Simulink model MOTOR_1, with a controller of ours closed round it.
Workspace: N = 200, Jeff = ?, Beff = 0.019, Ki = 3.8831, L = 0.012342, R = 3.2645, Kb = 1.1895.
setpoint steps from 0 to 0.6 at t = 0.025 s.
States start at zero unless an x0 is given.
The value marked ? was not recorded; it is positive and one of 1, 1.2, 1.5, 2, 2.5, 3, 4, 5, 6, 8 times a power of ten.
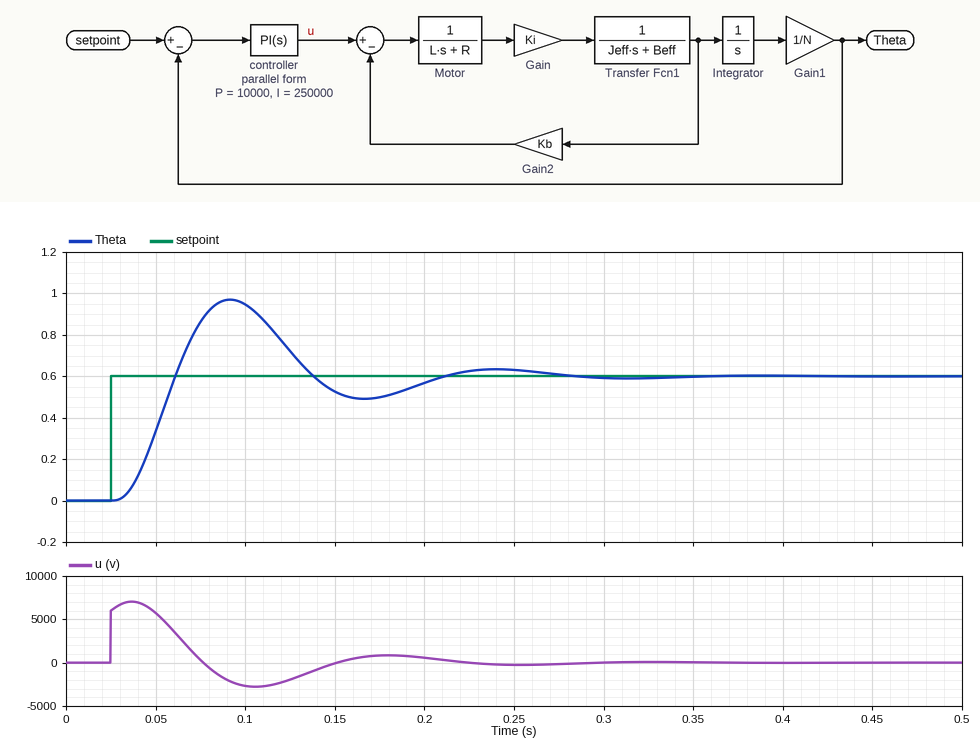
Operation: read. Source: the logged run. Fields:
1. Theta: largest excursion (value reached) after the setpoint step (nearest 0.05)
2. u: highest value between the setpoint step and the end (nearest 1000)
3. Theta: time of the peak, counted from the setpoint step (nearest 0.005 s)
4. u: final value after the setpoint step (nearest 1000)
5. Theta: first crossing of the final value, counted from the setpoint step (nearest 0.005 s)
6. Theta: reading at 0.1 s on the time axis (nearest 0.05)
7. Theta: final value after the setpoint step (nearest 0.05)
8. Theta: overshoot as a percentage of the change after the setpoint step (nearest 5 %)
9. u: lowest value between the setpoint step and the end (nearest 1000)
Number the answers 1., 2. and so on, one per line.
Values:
1. 0.95
2. 7000
3. 0.065 s
4. 0
5. 0.035 s
6. 0.95
7. 0.60
8. 60 %
9. -3000
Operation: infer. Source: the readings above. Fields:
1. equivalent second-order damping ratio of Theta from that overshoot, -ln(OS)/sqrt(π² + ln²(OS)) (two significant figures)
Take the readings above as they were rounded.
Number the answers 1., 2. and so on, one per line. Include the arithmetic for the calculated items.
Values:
1. ln(0.6) = -0.511; 0.511 / sqrt(9.870 + 0.261) = 0.16
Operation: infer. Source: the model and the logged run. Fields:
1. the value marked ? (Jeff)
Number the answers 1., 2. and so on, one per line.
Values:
1. 0.02
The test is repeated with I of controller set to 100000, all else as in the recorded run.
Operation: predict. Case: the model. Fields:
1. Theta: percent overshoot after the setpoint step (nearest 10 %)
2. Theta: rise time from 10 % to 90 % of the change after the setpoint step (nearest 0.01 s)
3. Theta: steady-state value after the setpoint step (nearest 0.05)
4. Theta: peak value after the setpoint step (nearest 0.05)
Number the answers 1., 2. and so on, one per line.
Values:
1. 30 %
2. 0.03 s
3. 0.60
4. 0.80
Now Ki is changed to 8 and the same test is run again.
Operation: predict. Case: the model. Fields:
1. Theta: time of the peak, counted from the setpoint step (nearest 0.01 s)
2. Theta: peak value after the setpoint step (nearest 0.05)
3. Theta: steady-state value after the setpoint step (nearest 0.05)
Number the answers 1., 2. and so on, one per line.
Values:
1. 0.06 s
2. 0.80
3. 0.60
